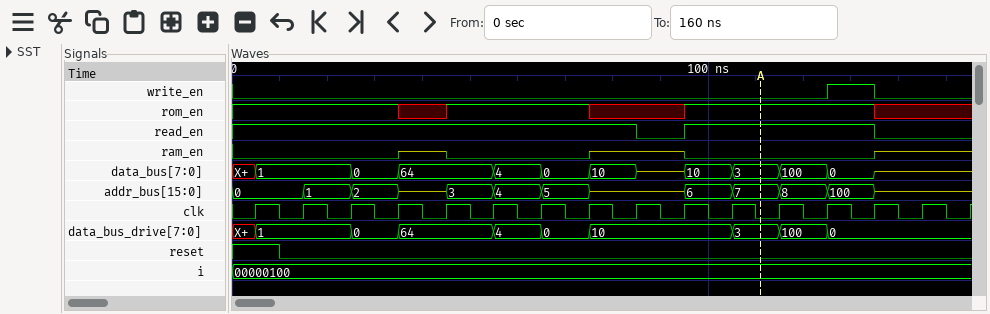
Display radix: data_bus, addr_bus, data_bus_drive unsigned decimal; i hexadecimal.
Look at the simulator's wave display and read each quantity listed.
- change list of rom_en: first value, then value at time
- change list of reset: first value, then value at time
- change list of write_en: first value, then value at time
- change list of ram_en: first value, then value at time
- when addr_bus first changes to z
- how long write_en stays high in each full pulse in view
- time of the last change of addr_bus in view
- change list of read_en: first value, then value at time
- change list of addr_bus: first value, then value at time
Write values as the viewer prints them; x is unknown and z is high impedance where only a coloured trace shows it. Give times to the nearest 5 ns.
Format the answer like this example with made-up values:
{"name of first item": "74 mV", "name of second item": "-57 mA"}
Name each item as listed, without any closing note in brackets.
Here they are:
{"change list of rom_en: first value, then value at time": "1, x at 35 ns, 1 at 45 ns, x at 75 ns, 1 at 95 ns, x at 135 ns", "change list of reset: first value, then value at time": "1, 0 at 10 ns", "change list of write_en: first value, then value at time": "0, 1 at 125 ns, 0 at 135 ns", "change list of ram_en: first value, then value at time": "0, z at 35 ns, 0 at 45 ns, z at 75 ns, 0 at 95 ns, z at 135 ns", "when addr_bus first changes to z": "35 ns", "how long write_en stays high in each full pulse in view": "10 ns", "time of the last change of addr_bus in view": "135 ns", "change list of read_en: first value, then value at time": "1, 0 at 85 ns, 1 at 95 ns, 0 at 135 ns", "change list of addr_bus: first value, then value at time": "0, 1 at 15 ns, 2 at 25 ns, z at 35 ns, 3 at 45 ns, 4 at 55 ns, 5 at 65 ns, z at 75 ns, 6 at 95 ns, 7 at 105 ns, 8 at 115 ns, 100 at 125 ns, z at 135 ns"}
